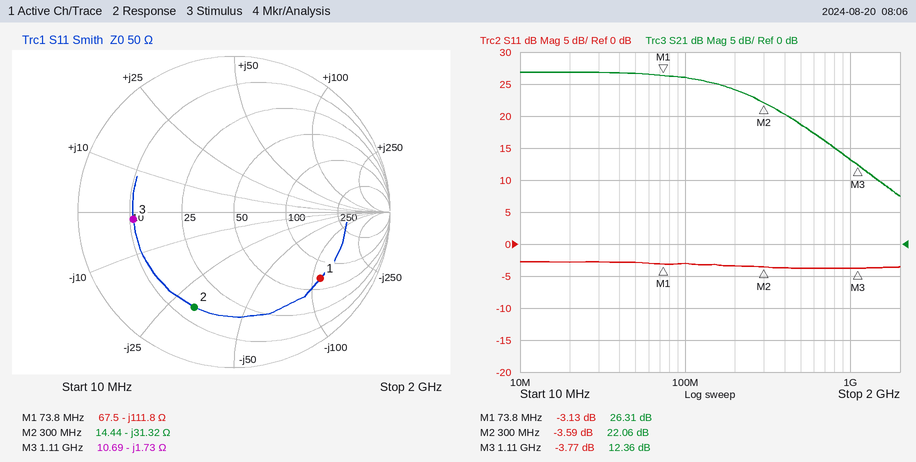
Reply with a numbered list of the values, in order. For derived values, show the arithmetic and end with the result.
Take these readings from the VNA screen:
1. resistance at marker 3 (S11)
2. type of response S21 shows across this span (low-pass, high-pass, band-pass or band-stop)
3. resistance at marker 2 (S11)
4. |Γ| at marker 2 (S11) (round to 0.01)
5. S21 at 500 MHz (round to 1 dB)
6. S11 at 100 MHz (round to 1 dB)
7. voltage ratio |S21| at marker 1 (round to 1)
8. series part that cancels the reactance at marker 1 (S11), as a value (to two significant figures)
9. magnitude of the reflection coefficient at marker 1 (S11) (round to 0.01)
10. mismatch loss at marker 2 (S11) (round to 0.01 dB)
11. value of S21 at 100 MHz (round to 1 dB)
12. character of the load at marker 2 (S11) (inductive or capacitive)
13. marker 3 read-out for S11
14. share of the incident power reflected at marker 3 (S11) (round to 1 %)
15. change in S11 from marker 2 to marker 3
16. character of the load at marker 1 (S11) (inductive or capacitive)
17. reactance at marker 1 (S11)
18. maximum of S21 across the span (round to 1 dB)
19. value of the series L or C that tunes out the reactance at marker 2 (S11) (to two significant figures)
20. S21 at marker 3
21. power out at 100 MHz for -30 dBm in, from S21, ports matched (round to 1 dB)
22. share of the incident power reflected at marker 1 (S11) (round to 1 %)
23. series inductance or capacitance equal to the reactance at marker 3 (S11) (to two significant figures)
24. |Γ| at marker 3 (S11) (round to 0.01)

1. 10.69 Ω
2. low-pass
3. 14.44 Ω
4. 0.66
5. 19 dB
6. -3 dB
7. 10^(26.31/20) ≈ 21
8. L = 111.8 Ω/(2π × 73.8 MHz) ≈ 241 nH, so 240 nH to two significant figures
9. 0.70
10. −10 log10(1 − 10^(-3.59/10)) ≈ 2.50 dB
11. 26 dB
12. capacitive
13. -3.77 dB
14. 10^(-3.77/10) ≈ 42 %
15. -3.77 − (-3.59) = -0.18 dB
16. capacitive
17. -111.8 Ω
18. 27 dB
19. L = 31.32 Ω/(2π × 300 MHz) ≈ 17 nH
20. 12.36 dB
21. -30 dBm + (26 dB) = -4 dBm
22. 10^(-3.13/10) ≈ 49 %
23. C = 1/(2π × 1.11 GHz × 1.73 Ω) ≈ 83 pF
24. 0.65
